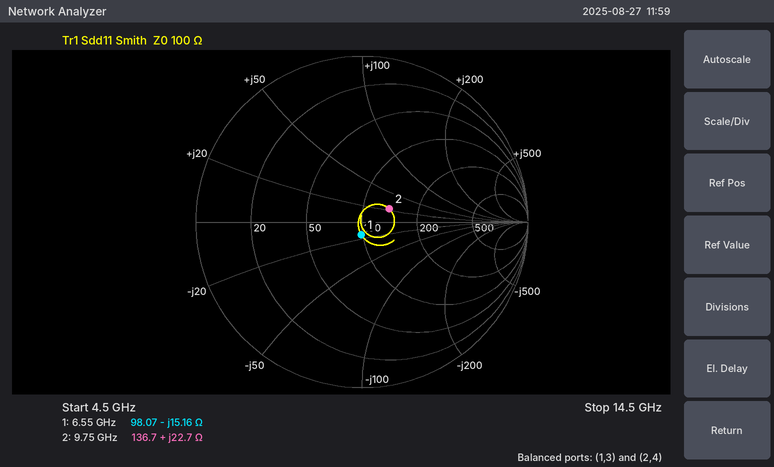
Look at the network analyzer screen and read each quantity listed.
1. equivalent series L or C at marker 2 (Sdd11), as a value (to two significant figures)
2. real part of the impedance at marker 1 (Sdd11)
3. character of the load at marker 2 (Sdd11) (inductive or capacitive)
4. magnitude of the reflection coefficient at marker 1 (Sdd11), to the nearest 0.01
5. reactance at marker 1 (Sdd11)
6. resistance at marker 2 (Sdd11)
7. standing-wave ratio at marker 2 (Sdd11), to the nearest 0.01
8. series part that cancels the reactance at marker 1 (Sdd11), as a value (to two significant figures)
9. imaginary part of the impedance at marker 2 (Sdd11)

370 pH
98.07 Ω
inductive
0.08
-15.16 Ω
136.7 Ω
1.44
370 pH
+22.7 Ω
